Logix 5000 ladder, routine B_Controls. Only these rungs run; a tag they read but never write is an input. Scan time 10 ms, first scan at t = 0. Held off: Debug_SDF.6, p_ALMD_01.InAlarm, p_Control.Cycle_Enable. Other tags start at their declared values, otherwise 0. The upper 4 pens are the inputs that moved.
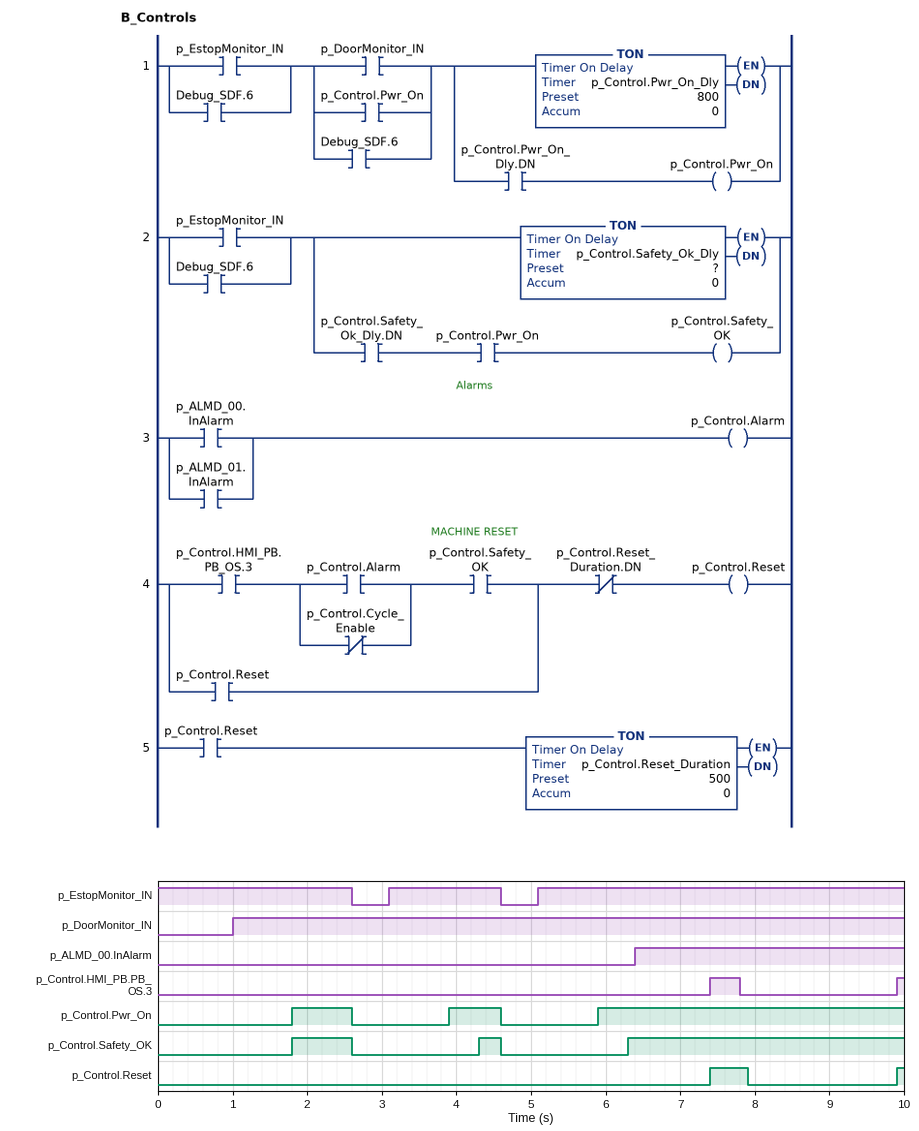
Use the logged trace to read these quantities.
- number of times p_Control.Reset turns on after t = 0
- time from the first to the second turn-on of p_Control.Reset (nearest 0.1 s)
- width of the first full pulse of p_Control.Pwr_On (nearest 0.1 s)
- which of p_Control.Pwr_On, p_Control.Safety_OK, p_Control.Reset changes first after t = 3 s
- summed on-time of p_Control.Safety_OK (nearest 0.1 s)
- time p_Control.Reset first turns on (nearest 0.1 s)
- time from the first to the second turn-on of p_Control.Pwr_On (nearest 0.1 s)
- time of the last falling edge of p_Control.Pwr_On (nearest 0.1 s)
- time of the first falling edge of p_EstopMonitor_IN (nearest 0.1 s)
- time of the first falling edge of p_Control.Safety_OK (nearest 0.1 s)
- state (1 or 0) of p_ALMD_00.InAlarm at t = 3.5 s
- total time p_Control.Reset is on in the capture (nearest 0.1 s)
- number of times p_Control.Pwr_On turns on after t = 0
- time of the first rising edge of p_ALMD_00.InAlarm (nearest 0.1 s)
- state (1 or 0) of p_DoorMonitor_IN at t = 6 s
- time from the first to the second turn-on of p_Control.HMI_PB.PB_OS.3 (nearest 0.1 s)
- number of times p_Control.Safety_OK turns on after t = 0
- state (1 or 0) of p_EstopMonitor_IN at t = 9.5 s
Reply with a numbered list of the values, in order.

1. 2
2. 2.5 s
3. 0.8 s
4. p_Control.Pwr_On
5. 4.8 s
6. 7.4 s
7. 2.1 s
8. 4.6 s
9. 2.6 s
10. 2.6 s
11. 0
12. 0.6 s
13. 3
14. 6.4 s
15. 1
16. 2.5 s
17. 3
18. 1
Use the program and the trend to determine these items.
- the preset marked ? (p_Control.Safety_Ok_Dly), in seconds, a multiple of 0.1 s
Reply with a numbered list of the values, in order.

1. 1.2 s
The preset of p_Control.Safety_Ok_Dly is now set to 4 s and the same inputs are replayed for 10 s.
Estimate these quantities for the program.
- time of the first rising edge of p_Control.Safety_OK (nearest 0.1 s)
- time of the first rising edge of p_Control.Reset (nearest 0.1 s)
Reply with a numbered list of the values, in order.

1. 9.1 s
2. 9.9 s
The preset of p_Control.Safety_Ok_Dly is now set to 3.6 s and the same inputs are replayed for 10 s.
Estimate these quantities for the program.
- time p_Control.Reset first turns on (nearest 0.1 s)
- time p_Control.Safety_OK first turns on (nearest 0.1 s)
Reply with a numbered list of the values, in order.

1. 9.9 s
2. 8.7 s
